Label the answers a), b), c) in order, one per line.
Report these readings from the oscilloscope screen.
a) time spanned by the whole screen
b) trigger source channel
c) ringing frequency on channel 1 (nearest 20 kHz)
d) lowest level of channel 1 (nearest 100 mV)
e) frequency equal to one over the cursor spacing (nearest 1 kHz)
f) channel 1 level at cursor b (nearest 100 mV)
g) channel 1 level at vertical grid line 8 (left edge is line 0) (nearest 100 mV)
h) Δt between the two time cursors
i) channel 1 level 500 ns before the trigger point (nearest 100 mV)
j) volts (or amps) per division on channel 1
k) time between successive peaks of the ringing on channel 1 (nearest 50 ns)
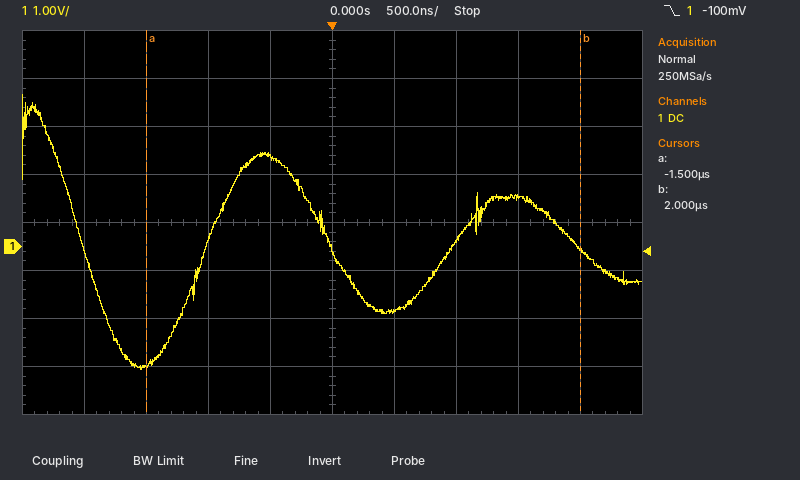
a) 5 µs
b) channel 1
c) 520 kHz
d) -2.6 V
e) 286 kHz
f) -100 mV
g) 1.0 V
h) 3.50 µs
i) 1.9 V
j) 1 V
k) 1.95 µs
